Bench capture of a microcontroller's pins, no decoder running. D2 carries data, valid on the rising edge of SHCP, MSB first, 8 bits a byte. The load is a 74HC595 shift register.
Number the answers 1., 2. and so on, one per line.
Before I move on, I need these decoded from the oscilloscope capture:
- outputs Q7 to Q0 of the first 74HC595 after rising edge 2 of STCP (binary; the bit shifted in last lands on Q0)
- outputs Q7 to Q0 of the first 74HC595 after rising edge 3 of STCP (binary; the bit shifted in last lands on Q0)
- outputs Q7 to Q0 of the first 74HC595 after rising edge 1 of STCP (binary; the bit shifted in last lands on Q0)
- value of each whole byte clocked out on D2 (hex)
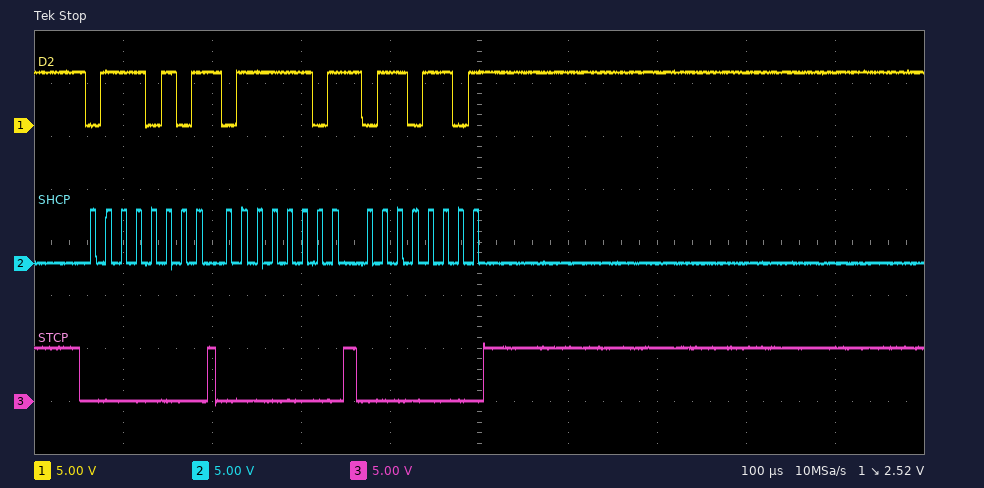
1. 01111101
2. 01101101
3. 01110101
4. 75 7D 6D
